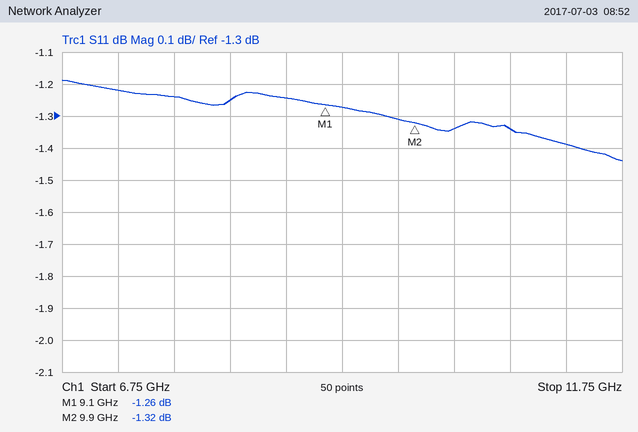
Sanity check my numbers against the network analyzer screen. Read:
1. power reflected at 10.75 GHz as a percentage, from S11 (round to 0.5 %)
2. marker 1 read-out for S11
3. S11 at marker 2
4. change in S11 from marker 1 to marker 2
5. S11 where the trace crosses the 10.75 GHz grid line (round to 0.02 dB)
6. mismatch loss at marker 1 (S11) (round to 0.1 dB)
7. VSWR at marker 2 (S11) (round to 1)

73.5 %
-1.26 dB
-1.32 dB
-0.06 dB
-1.34 dB
6.0 dB
13
